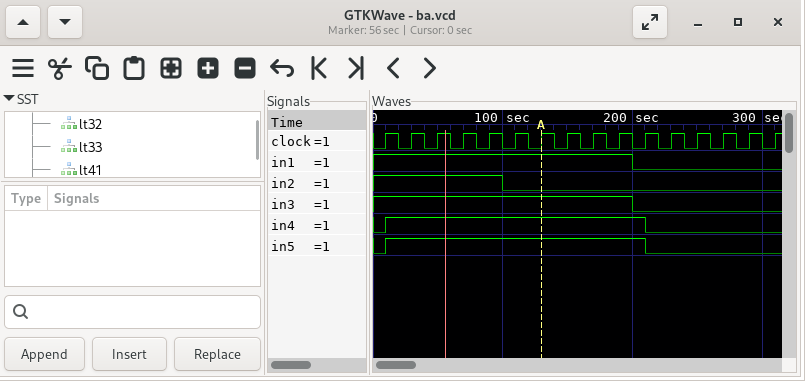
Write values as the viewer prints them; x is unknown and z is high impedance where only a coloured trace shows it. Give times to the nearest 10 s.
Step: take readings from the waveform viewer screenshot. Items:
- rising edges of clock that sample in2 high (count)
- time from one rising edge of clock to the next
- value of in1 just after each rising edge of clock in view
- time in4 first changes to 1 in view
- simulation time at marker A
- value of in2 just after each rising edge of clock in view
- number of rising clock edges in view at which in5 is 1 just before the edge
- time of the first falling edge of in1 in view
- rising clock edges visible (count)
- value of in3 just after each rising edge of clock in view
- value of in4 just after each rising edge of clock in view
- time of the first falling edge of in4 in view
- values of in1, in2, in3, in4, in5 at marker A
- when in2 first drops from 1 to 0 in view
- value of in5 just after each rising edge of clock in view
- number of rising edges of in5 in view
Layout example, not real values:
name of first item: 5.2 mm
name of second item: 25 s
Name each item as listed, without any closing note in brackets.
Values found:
rising edges of clock that sample in2 high: 5
time from one rising edge of clock to the next: 20 s
value of in1 just after each rising edge of clock in view: 1 1 1 1 1 1 1 1 1 1 0 0 0 0 0 0
time in4 first changes to 1 in view: 10 s
simulation time at marker A: 130 s
value of in2 just after each rising edge of clock in view: 1 1 1 1 1 0 0 0 0 0 0 0 0 0 0 0
number of rising clock edges in view at which in5 is 1 just before the edge: 10
time of the first falling edge of in1 in view: 200 s
rising clock edges visible: 16
value of in3 just after each rising edge of clock in view: 1 1 1 1 1 1 1 1 1 1 0 0 0 0 0 0
value of in4 just after each rising edge of clock in view: 1 1 1 1 1 1 1 1 1 1 0 0 0 0 0 0
time of the first falling edge of in4 in view: 210 s
values of in1, in2, in3, in4, in5 at marker A: in1=1, in2=0, in3=1, in4=1, in5=1
when in2 first drops from 1 to 0 in view: 100 s
value of in5 just after each rising edge of clock in view: 1 1 1 1 1 1 1 1 1 1 0 0 0 0 0 0
number of rising edges of in5 in view: 1
